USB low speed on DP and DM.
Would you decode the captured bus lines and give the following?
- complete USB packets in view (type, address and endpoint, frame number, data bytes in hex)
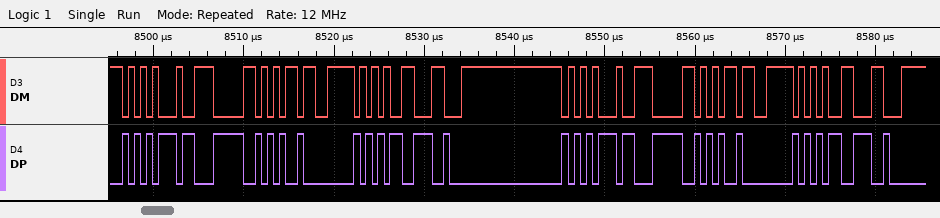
IN ADDR 47 EP 0, NAK, IN ADDR 47 EP 0, NAK
